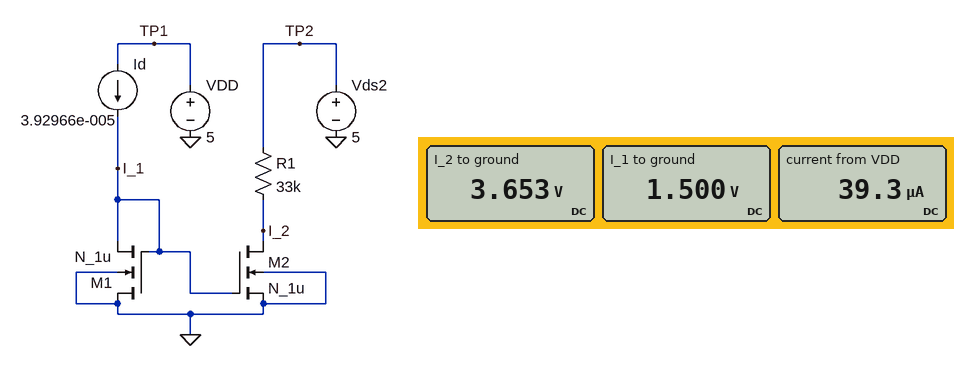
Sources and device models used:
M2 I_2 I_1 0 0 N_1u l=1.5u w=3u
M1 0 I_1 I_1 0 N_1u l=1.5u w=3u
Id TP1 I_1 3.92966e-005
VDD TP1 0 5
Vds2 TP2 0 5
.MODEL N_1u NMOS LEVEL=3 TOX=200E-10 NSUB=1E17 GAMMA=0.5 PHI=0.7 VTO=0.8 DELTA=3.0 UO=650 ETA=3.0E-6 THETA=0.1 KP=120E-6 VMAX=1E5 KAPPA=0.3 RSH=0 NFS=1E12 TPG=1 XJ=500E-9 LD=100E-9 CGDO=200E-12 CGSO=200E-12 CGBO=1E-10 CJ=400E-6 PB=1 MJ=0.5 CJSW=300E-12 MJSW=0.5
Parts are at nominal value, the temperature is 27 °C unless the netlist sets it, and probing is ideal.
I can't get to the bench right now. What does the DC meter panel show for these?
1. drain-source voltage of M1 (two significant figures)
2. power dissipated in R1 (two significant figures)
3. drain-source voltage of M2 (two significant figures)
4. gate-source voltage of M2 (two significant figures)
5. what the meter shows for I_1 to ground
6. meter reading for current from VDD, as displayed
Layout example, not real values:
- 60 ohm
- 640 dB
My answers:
- -1.5 V
- 55 µW
- 3.7 V
- 1.5 V
- 1.500 V
- 39.3 µA
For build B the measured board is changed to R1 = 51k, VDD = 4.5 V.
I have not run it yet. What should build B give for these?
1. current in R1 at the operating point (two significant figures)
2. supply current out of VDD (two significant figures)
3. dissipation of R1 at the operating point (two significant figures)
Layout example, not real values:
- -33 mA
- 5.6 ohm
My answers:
- 40 µA
- 39 µA
- 83 µW
